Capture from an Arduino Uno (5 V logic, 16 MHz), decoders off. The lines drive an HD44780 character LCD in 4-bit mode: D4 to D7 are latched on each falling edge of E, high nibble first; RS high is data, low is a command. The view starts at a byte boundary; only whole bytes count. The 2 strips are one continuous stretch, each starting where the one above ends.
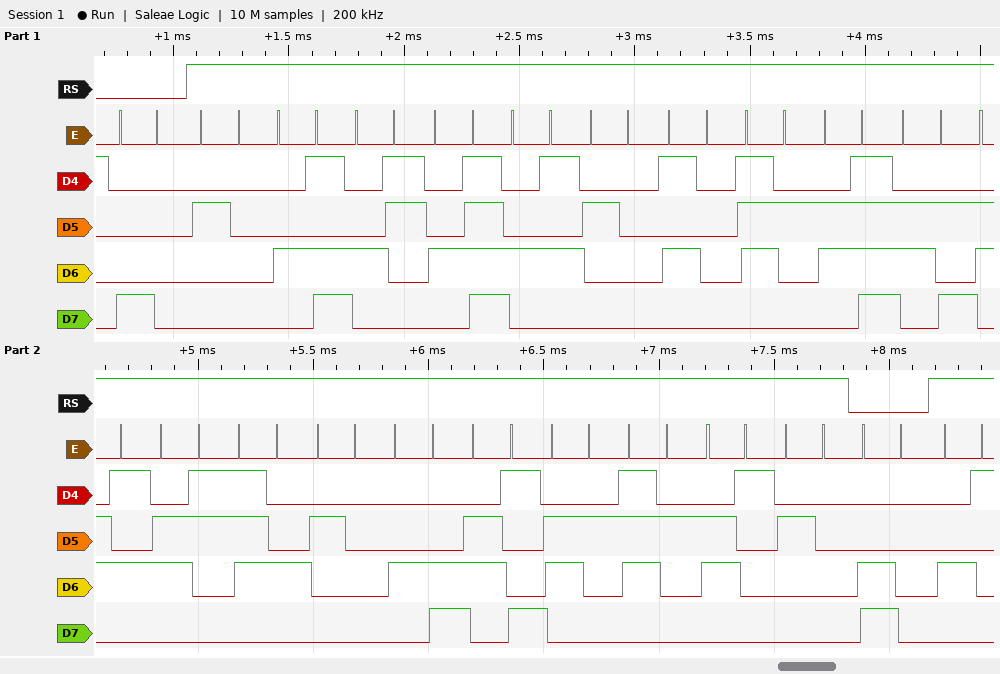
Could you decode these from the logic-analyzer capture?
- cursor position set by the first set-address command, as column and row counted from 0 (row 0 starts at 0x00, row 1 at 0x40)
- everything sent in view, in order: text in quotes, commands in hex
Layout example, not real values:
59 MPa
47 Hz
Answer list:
column 0, row 0
0x80 " MCOE Project Libra " 0xC0 "A"
